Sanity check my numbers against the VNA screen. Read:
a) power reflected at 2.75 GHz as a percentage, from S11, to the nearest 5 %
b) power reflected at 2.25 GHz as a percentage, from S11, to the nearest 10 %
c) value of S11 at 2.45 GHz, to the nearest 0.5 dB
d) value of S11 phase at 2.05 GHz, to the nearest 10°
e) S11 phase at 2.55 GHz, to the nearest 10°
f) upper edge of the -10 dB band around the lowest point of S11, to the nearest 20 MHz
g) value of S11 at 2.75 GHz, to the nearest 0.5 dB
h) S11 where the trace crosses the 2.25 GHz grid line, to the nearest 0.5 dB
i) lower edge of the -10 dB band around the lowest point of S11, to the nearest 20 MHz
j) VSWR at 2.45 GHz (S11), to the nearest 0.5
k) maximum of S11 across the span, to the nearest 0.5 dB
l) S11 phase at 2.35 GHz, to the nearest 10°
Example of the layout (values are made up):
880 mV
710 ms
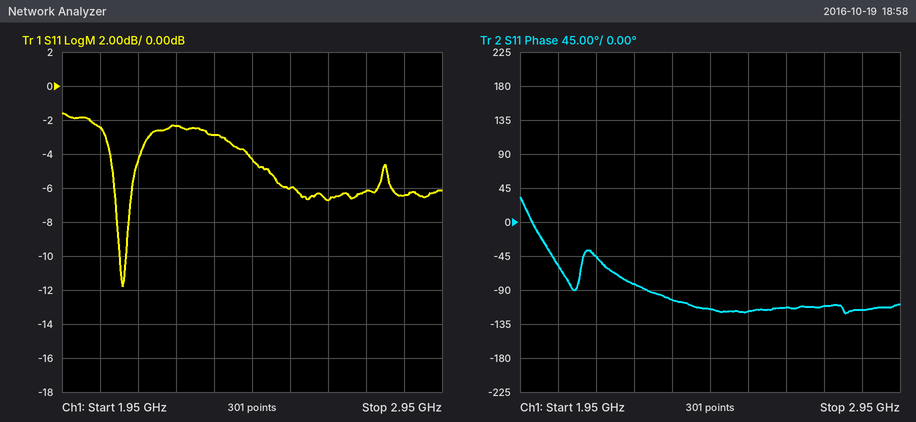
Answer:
25 %
60 %
-4.5 dB
-60°
-120°
2.12 GHz
-6.0 dB
-2.5 dB
2.10 GHz
4.0
-1.5 dB
-100°
